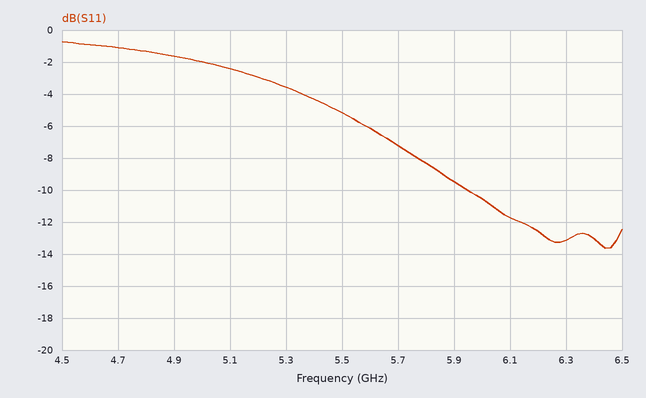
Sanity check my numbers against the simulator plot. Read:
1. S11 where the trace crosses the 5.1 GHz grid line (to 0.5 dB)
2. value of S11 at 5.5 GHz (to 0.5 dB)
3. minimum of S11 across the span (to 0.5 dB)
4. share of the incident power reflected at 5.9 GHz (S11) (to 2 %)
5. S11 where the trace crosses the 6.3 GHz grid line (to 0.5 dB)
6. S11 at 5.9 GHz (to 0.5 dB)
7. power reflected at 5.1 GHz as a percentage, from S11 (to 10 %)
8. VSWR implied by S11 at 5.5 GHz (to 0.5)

-2.5 dB
-5.0 dB
-13.5 dB
12 %
-13.0 dB
-9.5 dB
60 %
3.5
